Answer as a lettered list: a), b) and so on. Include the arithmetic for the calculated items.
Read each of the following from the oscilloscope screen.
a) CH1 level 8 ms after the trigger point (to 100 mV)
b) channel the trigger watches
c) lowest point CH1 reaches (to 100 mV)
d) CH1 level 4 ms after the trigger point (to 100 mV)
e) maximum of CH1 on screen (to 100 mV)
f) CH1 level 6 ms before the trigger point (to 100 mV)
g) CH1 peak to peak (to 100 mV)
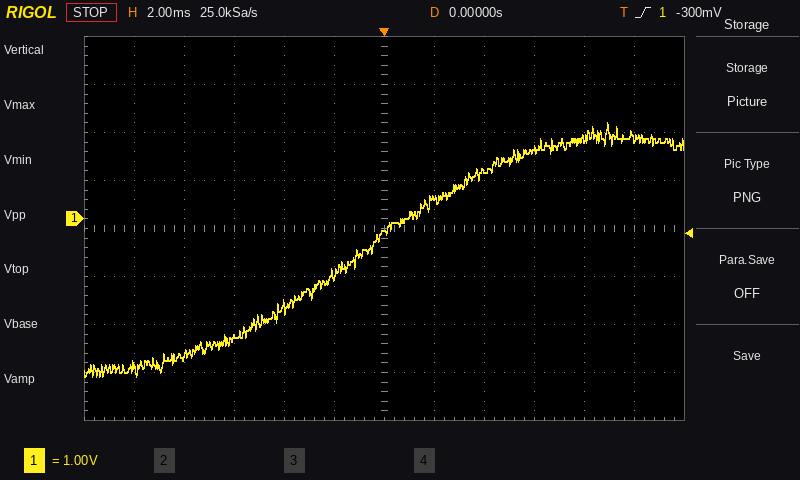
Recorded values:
a) 1.7 V
b) CH1
c) -3.3 V
d) 1.0 V
e) 2.0 V
f) -2.5 V
g) 2.0 V − (-3.3 V) = 5.3 V
